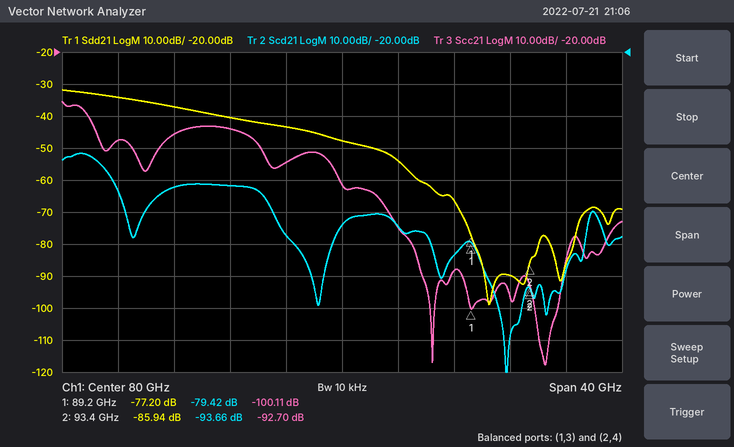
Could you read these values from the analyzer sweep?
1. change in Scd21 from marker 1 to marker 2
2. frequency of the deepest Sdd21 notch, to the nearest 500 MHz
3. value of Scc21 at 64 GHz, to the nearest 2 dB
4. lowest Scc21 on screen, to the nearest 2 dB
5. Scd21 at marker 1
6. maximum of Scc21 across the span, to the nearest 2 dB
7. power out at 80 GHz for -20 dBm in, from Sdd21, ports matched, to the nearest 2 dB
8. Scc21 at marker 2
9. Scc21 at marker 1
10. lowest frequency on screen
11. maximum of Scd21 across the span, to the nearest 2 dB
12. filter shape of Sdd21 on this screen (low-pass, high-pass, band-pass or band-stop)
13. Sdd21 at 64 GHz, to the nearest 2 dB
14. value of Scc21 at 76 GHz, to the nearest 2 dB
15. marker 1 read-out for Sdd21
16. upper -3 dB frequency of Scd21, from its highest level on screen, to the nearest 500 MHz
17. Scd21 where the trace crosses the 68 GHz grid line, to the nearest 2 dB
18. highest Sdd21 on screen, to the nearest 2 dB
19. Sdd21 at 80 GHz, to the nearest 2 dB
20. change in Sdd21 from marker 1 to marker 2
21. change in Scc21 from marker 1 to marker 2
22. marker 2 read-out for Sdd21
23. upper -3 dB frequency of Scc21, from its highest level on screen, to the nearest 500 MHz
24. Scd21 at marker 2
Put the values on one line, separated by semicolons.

-14.24 dB; 90.5 GHz; -48 dB; -118 dB; -79.42 dB; -36 dB; -68 dBm; -92.70 dB; -100.11 dB; 60 GHz; -52 dB; low-pass; -34 dB; -54 dB; -77.20 dB; 62.5 GHz; -62 dB; -32 dB; -48 dB; -8.74 dB; 7.41 dB; -85.94 dB; 61.5 GHz; -93.66 dB
